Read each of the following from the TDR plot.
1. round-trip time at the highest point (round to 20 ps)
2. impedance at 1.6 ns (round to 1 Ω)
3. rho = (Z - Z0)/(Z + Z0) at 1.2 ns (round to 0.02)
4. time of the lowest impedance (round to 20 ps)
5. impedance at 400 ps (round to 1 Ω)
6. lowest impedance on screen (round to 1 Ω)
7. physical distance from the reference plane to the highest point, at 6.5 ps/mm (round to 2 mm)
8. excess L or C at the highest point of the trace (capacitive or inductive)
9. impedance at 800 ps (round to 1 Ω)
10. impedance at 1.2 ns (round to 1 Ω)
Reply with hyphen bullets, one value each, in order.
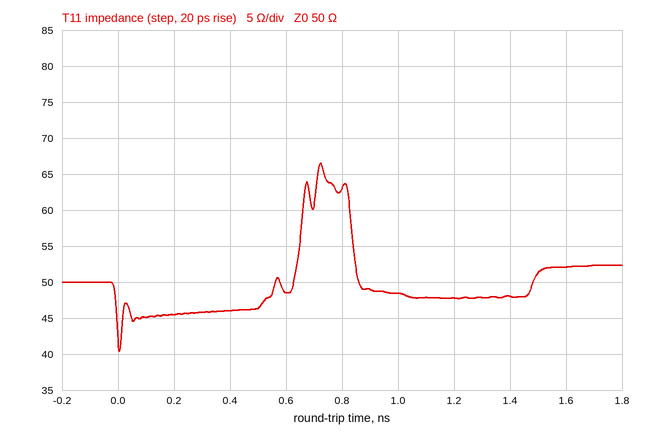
- 720 ps
- 52 Ω
- -0.02
- 0 ps
- 46 Ω
- 40 Ω
- 56 mm
- inductive
- 63 Ω
- 48 Ω
